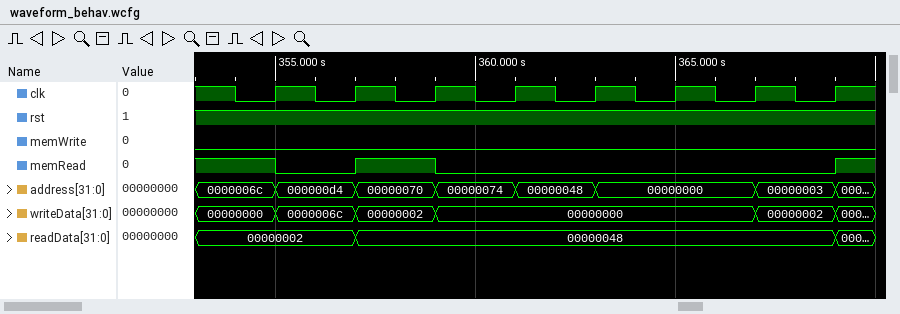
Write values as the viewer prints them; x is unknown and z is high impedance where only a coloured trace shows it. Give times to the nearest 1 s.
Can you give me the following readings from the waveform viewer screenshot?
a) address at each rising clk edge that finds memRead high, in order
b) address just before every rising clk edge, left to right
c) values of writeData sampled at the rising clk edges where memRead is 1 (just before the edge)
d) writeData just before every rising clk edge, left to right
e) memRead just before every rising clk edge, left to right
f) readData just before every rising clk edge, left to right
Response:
0000006c, 00000070
0000006c, 000000d4, 00000070, 00000074, 00000048, 00000000, 00000000, 00000003
00000000, 00000002
00000000, 0000006c, 00000002, 00000000, 00000000, 00000000, 00000000, 00000002
1 0 1 0 0 0 0 0
00000002, 00000002, 00000048, 00000048, 00000048, 00000048, 00000048, 00000048
